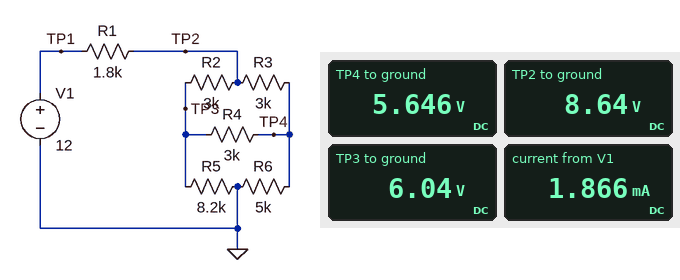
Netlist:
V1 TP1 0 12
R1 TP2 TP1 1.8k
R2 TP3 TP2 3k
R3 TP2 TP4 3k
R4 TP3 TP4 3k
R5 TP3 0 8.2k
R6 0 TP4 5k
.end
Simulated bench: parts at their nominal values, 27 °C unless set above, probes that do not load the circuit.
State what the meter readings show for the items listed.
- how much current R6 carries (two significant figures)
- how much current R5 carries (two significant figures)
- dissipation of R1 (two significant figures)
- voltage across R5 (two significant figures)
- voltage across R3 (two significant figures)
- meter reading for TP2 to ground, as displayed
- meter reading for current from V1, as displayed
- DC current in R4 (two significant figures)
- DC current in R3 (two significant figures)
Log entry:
1.1 mA
740 µA
6.3 mW
6.0 V
3.0 V
8.64 V
1.866 mA
130 µA
1.0 mA
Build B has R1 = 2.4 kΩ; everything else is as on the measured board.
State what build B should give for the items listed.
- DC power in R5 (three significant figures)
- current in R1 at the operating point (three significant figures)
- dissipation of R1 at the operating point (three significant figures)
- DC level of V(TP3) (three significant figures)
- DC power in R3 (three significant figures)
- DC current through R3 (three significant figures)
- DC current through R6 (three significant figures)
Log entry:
3.72 mW
1.71 mA
6.99 mW
5.52 V
2.50 mW
913 µA
1.03 mA
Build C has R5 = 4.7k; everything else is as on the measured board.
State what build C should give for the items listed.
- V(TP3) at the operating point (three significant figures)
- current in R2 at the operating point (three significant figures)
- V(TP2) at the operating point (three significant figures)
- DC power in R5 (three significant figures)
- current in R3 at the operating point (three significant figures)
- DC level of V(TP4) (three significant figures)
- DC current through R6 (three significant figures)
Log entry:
5.05 V
1.06 mA
8.23 V
5.43 mW
1.04 mA
5.11 V
1.02 mA
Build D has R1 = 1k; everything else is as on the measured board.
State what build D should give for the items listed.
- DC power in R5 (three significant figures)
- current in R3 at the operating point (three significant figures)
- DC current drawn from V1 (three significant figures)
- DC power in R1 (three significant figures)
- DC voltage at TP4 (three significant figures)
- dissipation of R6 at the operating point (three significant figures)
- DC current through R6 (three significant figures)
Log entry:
5.80 mW
1.14 mA
2.13 mA
4.54 mW
6.45 V
8.32 mW
1.29 mA
